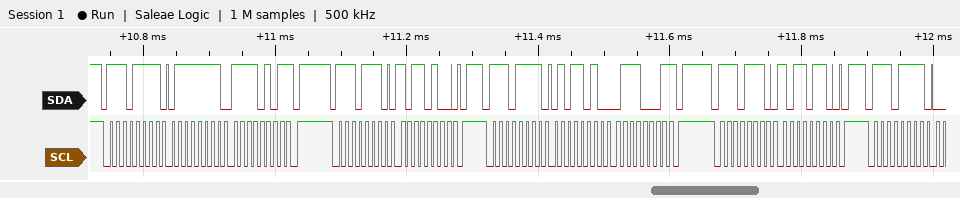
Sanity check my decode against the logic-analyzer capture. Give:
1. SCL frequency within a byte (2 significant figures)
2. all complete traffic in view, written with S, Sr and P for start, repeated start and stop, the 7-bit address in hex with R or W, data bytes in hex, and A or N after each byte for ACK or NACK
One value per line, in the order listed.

100 kHz
S 77R A 7F A F5 N P S 77W A B4 A P S 77R A 5A A 71 N P S 77W A B6 A P S 77R A
